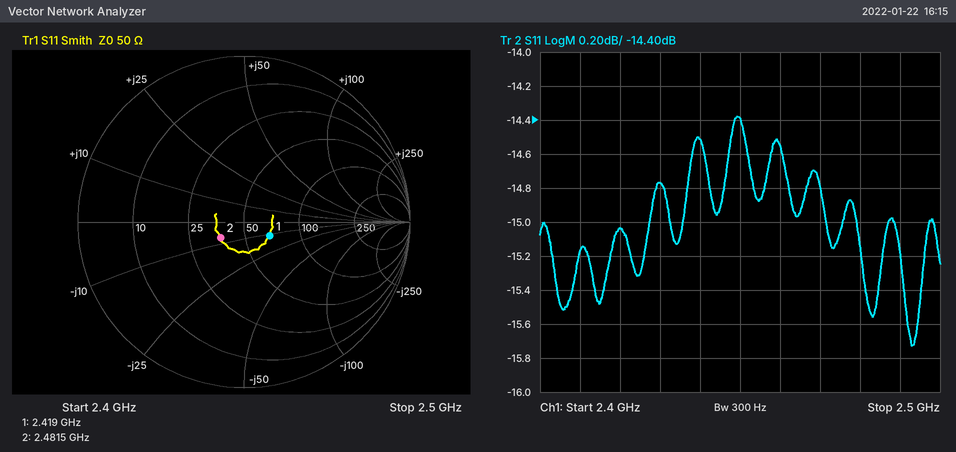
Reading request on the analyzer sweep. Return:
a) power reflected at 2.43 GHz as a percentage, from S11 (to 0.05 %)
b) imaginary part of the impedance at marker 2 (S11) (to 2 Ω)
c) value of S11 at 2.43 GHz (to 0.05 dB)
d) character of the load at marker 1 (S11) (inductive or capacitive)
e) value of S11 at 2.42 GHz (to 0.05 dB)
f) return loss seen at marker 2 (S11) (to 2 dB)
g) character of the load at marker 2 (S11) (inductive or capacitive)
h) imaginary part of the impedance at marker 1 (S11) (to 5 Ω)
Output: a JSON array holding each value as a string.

["3.35 %", "-8 Ω", "-14.75 dB", "capacitive", "-15.05 dB", "16 dB", "capacitive", "-10 Ω"]
